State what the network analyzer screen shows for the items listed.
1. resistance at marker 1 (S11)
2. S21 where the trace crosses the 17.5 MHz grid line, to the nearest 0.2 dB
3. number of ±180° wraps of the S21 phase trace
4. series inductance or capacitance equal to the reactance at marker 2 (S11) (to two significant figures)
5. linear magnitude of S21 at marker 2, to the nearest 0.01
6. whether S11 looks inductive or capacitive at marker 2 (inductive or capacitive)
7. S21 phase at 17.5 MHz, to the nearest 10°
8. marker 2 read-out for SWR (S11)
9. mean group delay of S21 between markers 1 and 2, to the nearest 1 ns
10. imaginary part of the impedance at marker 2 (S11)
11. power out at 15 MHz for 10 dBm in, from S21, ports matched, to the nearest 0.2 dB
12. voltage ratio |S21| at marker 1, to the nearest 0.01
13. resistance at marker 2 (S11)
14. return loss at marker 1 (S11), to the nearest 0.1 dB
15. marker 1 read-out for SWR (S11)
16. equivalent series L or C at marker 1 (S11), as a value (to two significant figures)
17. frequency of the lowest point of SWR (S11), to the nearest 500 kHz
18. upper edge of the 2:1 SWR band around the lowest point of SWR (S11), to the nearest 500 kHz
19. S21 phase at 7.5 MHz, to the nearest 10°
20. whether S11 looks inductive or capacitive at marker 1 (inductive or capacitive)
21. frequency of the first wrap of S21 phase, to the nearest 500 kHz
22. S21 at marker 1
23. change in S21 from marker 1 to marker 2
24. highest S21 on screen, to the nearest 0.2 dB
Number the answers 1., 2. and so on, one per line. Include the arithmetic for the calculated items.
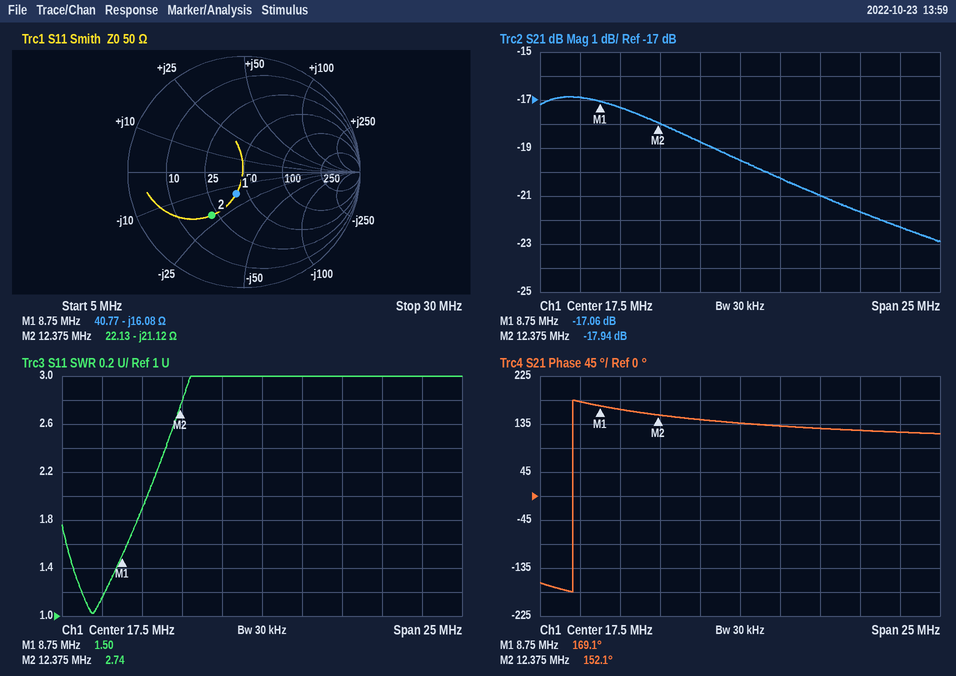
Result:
1. 40.77 Ω
2. -19.6 dB
3. 1
4. C = 1/(2π × 12.375 MHz × 21.12 Ω) ≈ 609 pF, so 610 pF to two significant figures
5. 10^(-17.94/20) ≈ 0.13
6. capacitive
7. 140°
8. 2.74
9. −(152.1° − (169.1°))/(360° × 3.625 MHz) ≈ 13 ns
10. -21.12 Ω
11. 10 dBm + (-18.8 dB) = -8.8 dBm
12. 10^(-17.06/20) ≈ 0.14
13. 22.13 Ω
14. 13.9 dB
15. 1.50
16. C = 1/(2π × 8.75 MHz × 16.08 Ω) ≈ 1.1 nF
17. 7.0 MHz
18. 10.5 MHz
19. 180°
20. capacitive
21. 7.0 MHz
22. -17.06 dB
23. -17.94 − (-17.06) = -0.88 dB
24. -16.8 dB
